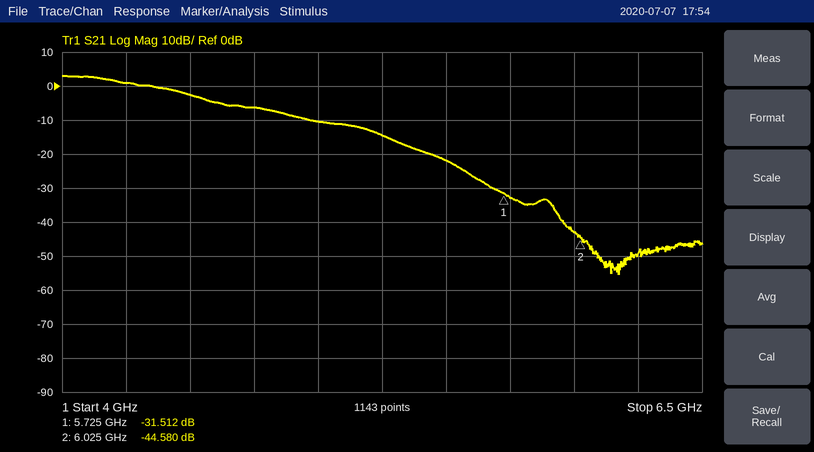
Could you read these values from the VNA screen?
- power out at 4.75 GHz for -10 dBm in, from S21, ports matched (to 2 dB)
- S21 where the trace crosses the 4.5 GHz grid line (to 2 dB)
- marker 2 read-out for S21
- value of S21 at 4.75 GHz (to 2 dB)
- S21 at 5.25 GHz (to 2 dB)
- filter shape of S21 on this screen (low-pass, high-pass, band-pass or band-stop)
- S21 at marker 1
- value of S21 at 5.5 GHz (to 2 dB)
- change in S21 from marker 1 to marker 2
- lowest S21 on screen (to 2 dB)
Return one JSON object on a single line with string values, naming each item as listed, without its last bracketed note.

{"power out at 4.75 GHz for -10 dBm in, from S21, ports matched": "-16 dBm", "S21 where the trace crosses the 4.5 GHz grid line": "-2 dB", "marker 2 read-out for S21": "-44.580 dB", "value of S21 at 4.75 GHz": "-6 dB", "S21 at 5.25 GHz": "-14 dB", "filter shape of S21 on this screen": "low-pass", "S21 at marker 1": "-31.512 dB", "value of S21 at 5.5 GHz": "-22 dB", "change in S21 from marker 1 to marker 2": "-13.068 dB", "lowest S21 on screen": "-56 dB"}
